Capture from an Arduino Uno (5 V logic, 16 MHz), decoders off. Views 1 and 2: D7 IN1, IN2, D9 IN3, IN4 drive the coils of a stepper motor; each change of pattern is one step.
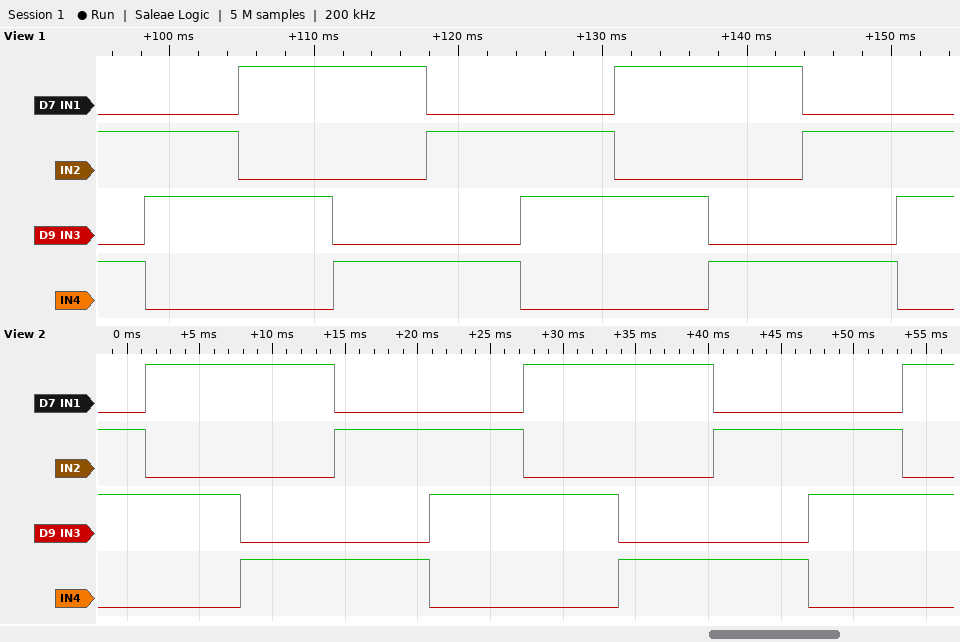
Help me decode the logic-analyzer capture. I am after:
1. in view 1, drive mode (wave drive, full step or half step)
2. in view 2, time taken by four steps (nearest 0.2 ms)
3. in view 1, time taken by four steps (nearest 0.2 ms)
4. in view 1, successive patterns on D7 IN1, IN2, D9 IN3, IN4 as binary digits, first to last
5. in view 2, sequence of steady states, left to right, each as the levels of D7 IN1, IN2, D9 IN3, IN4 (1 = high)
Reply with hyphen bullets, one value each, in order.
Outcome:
- full step
- 26.0 ms
- 26.0 ms
- 0101 0110 1010 1001 0101 0110 1010 1001 0101 0110
- 0110 1010 1001 0101 0110 1010 1001 0101 0110 1010
